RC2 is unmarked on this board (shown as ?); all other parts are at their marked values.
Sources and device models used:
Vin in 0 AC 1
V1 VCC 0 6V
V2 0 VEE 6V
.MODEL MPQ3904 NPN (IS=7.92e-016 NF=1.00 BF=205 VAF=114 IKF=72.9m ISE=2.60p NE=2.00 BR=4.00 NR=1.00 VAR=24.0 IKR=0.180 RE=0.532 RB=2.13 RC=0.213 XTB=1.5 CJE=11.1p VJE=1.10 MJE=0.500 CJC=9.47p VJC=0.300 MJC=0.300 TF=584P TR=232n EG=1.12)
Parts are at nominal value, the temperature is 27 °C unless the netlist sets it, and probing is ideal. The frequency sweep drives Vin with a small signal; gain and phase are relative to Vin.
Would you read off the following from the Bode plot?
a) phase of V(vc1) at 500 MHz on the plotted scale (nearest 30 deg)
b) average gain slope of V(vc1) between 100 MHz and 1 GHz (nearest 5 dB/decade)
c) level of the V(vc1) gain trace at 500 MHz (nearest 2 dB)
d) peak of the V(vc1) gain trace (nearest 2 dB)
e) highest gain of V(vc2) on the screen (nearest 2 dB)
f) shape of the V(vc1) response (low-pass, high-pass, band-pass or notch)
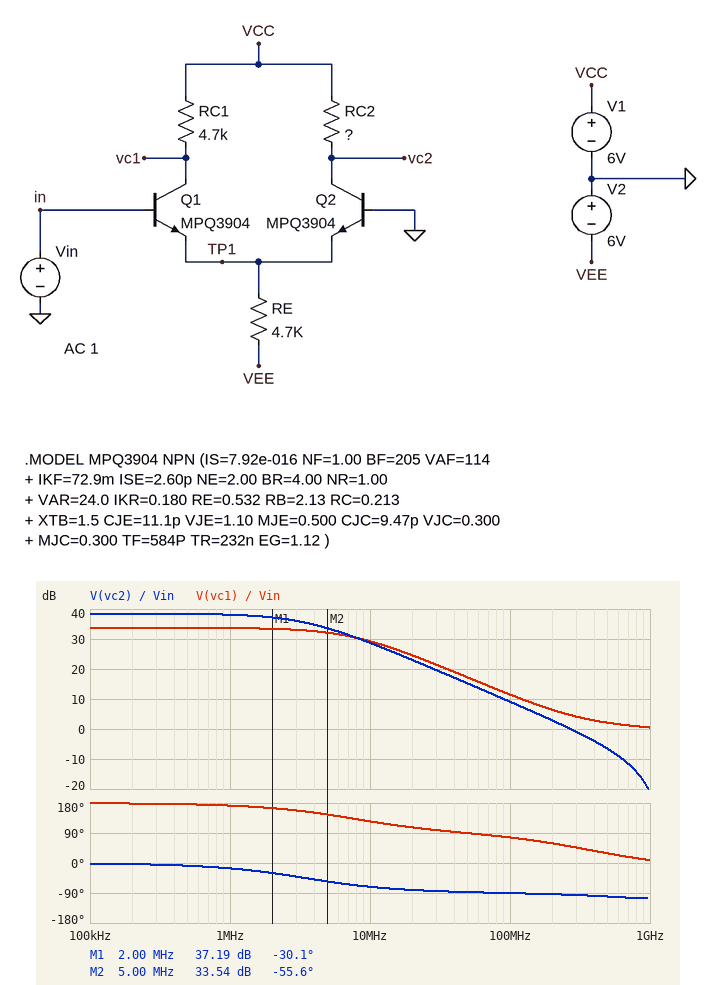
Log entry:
30 deg
-10 dB/decade
2 dB
34 dB
38 dB
low-pass
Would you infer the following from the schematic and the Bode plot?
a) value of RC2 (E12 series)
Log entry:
8.2 kΩ
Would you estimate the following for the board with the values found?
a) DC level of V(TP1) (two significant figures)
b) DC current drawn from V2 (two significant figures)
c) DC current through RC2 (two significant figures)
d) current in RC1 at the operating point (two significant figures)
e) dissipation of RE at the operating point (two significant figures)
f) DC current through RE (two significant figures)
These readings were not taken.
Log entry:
-710 mV
1.1 mA
550 µA
560 µA
6.0 mW
1.1 mA
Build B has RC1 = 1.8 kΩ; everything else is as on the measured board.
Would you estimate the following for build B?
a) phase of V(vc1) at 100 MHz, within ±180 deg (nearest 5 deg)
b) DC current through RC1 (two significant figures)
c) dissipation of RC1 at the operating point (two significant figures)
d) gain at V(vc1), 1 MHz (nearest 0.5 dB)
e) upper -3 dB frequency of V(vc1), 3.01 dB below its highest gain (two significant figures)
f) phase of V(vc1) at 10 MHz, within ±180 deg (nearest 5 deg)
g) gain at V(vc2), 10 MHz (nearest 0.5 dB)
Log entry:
85 deg
570 µA
580 µW
25.5 dB
22 MHz
155 deg
29.0 dB
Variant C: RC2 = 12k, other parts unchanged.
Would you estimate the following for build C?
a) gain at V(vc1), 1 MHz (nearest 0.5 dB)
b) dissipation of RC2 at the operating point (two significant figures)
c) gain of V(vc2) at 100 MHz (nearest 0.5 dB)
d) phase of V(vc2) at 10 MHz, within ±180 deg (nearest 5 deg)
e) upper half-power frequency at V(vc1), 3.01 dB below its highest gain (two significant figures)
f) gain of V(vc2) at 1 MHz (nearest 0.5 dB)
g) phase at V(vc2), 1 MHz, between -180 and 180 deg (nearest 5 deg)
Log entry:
33.0 dB
3.6 mW
-8.5 dB
-85 deg
8.2 MHz
30.5 dB
-60 deg
